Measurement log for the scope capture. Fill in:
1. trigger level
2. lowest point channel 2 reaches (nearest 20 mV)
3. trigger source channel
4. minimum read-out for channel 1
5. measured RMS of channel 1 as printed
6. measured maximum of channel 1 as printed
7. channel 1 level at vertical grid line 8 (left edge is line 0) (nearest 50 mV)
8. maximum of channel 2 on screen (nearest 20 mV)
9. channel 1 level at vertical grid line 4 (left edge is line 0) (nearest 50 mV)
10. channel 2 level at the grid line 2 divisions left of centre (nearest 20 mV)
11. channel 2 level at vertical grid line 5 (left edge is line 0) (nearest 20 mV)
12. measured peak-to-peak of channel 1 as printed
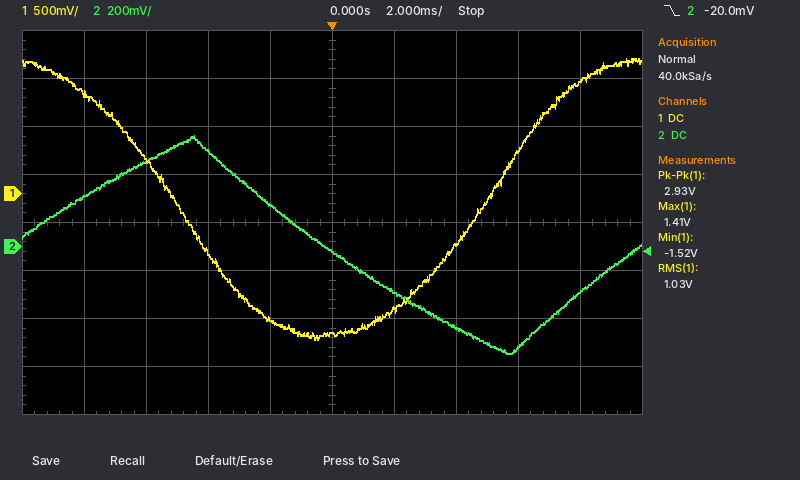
-20.0 mV
-440 mV
channel 2
-1.52 V
1.03 V
1.41 V
450 mV
460 mV
-1.30 V
400 mV
-20 mV
2.93 V
